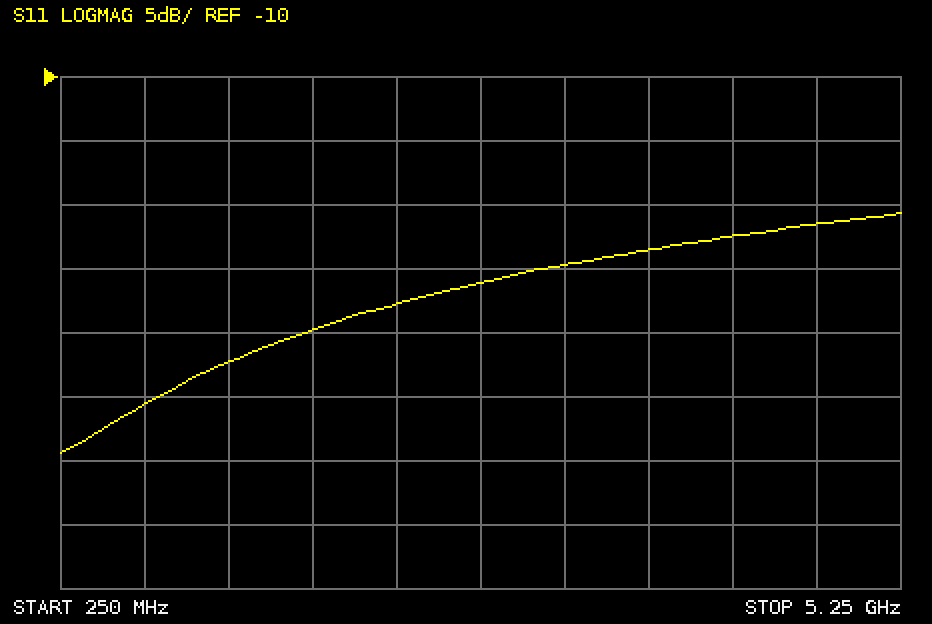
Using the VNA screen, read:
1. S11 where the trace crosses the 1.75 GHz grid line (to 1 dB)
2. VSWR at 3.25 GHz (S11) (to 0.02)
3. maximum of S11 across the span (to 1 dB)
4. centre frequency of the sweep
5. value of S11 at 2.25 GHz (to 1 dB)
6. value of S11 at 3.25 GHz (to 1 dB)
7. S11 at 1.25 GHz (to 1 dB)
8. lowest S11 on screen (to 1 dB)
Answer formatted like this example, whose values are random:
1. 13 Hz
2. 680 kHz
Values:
1. -30 dB
2. 1.12
3. -21 dB
4. 2.75 GHz
5. -28 dB
6. -25 dB
7. -32 dB
8. -39 dB
